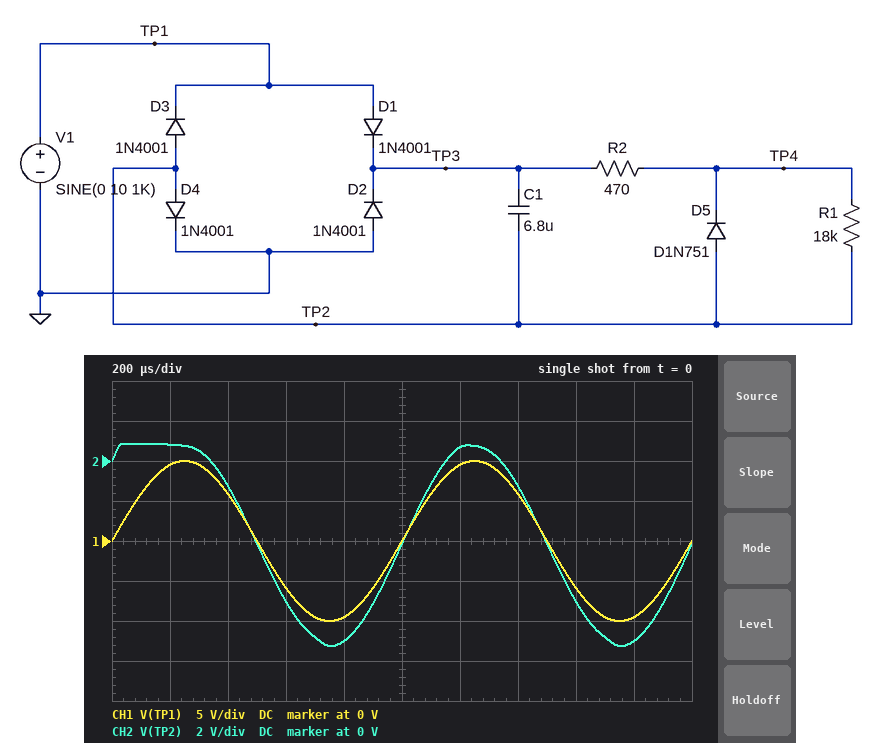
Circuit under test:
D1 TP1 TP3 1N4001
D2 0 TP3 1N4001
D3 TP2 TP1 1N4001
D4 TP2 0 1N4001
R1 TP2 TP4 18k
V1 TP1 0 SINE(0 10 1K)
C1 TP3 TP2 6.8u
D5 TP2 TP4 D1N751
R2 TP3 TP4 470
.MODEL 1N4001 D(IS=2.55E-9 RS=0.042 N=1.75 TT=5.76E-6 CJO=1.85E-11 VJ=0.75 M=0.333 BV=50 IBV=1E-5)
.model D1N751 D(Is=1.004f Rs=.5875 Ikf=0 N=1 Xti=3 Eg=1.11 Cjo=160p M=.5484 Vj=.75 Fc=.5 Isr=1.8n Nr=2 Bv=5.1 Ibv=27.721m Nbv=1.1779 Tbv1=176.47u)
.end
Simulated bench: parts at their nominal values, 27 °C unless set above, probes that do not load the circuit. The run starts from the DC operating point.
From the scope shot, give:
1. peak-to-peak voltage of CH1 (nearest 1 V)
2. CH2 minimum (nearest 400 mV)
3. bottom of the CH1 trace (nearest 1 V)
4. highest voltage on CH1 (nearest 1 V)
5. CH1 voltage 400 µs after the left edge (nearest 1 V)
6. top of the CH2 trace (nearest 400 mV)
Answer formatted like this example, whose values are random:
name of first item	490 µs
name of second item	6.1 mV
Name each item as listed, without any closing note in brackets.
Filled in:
peak-to-peak voltage of CH1	20 V
CH2 minimum	-9.2 V
bottom of the CH1 trace	-10 V
highest voltage on CH1	10 V
CH1 voltage 400 µs after the left edge	6 V
top of the CH2 trace	800 mV
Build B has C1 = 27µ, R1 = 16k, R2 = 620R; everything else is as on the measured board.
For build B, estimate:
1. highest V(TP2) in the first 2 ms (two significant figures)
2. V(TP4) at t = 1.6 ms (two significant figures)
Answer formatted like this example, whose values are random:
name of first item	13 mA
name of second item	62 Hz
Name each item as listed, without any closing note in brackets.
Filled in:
highest V(TP2) in the first 2 ms	980 mV
V(TP4) at t = 1.6 ms	-2.1 V
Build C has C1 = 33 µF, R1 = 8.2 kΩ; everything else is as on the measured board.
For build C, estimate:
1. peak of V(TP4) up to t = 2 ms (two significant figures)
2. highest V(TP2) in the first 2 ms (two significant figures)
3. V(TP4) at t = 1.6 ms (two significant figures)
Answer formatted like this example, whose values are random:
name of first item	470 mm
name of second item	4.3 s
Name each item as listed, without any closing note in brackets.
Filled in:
peak of V(TP4) up to t = 2 ms	6.0 V
highest V(TP2) in the first 2 ms	1.0 V
V(TP4) at t = 1.6 ms	-2.1 V
